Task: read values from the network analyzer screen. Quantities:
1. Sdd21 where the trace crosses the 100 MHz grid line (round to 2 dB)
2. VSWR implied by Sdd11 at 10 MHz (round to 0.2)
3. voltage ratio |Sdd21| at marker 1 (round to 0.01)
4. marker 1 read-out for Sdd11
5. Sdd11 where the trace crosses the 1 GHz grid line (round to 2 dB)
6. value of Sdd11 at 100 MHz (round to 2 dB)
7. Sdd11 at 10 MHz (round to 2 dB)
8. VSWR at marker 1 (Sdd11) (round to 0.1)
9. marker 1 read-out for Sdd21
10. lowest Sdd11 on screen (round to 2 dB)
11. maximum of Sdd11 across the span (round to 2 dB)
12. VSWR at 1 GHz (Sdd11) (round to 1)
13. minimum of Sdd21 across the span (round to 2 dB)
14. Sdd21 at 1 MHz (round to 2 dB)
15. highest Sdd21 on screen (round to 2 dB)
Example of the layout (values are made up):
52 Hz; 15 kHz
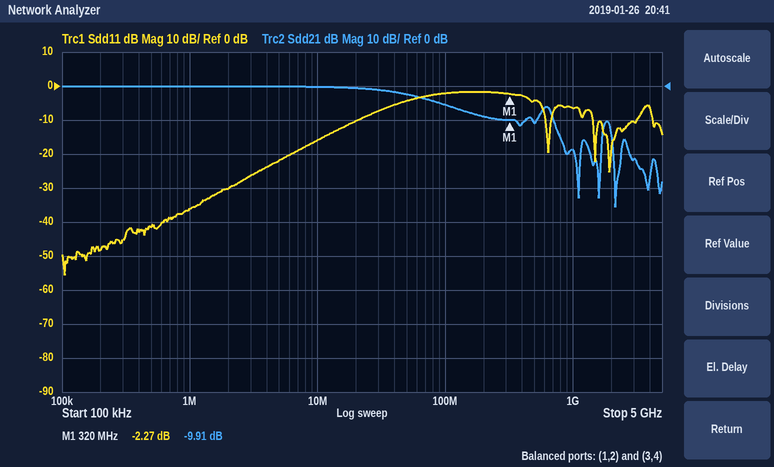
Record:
-6 dB; 1.4; 0.32; -2.27 dB; -6 dB; -2 dB; -16 dB; 7.7; -9.91 dB; -56 dB; -2 dB; 3; -36 dB; 0 dB; 0 dB
